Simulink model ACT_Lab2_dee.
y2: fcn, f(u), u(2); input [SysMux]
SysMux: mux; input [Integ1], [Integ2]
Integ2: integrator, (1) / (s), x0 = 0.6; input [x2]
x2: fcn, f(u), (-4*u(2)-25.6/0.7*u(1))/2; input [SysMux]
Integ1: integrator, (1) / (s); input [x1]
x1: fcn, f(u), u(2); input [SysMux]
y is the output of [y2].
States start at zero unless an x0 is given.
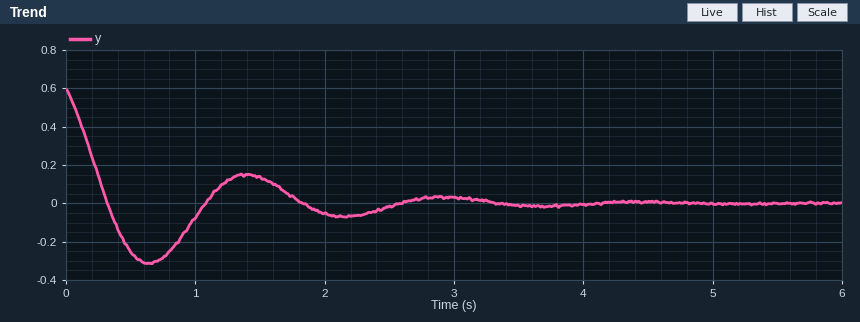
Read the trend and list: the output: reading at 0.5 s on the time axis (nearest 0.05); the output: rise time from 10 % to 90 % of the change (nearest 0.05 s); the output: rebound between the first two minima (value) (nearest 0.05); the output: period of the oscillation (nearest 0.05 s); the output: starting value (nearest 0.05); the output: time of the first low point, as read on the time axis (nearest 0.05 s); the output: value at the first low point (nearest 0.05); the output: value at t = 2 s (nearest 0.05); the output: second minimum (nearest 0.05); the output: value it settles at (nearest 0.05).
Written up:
-0.25
0.25 s
0.15
1.50 s
0.60
0.65 s
-0.30
-0.05
-0.05
0.00
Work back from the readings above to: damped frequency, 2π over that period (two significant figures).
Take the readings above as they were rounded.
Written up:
4.2 rad/s
